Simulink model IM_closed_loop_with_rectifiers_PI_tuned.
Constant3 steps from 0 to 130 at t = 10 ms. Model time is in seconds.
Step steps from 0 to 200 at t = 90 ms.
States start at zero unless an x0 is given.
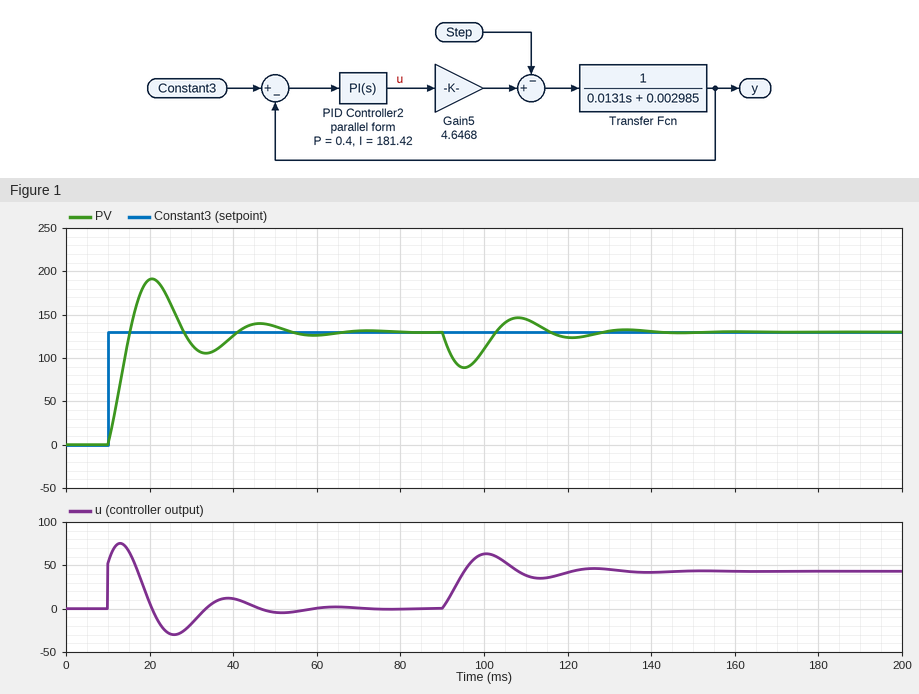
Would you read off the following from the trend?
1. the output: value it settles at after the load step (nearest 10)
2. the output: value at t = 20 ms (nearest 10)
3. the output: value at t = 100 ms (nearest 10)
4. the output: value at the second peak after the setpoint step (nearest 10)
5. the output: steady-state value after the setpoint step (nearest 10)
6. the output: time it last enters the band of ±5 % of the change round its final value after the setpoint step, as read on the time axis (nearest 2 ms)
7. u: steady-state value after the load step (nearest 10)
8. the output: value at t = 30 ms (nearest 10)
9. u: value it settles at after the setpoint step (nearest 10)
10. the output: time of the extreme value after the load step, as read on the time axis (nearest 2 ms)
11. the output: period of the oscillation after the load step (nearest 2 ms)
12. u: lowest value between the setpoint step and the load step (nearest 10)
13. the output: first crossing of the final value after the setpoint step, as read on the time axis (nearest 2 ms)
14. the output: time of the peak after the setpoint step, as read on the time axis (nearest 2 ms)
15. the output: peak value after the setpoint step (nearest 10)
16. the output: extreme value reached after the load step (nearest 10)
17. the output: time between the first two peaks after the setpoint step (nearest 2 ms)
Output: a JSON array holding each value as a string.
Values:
["130", "190", "110", "140", "130", "50 ms", "40", "120", "0", "96 ms", "26 ms", "-30", "16 ms", "20 ms", "190", "90", "26 ms"]
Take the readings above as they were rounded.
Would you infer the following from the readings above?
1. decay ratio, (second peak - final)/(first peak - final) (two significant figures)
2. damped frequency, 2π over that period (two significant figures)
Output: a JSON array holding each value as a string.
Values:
["0.17", "0.24 rad/ms"]
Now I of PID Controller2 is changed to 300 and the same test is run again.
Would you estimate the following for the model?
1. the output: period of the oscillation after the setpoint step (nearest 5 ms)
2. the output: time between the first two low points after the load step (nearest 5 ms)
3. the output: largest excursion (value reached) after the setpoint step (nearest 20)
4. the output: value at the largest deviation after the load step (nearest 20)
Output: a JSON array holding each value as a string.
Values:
["20 ms", "20 ms", "200", "100"]
